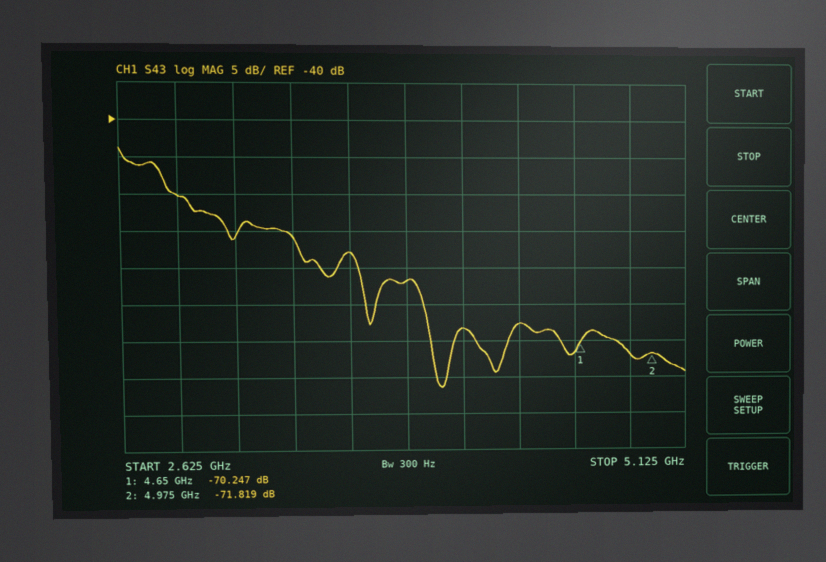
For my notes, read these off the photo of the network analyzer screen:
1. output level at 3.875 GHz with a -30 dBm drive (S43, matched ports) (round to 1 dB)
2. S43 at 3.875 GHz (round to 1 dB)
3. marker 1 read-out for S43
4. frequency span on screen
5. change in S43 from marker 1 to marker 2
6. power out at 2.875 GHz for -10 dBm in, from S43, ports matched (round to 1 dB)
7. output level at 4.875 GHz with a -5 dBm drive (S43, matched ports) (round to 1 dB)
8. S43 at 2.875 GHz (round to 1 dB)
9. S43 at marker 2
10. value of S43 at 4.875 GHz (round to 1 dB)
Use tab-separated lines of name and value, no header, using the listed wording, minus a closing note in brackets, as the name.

output level at 3.875 GHz with a -30 dBm drive (S43, matched ports)	-92 dBm
S43 at 3.875 GHz	-62 dB
marker 1 read-out for S43	-70.247 dB
frequency span on screen	2.5 GHz
change in S43 from marker 1 to marker 2	-1.572 dB
power out at 2.875 GHz for -10 dBm in, from S43, ports matched	-60 dBm
output level at 4.875 GHz with a -5 dBm drive (S43, matched ports)	-77 dBm
S43 at 2.875 GHz	-50 dB
S43 at marker 2	-71.819 dB
value of S43 at 4.875 GHz	-72 dB
